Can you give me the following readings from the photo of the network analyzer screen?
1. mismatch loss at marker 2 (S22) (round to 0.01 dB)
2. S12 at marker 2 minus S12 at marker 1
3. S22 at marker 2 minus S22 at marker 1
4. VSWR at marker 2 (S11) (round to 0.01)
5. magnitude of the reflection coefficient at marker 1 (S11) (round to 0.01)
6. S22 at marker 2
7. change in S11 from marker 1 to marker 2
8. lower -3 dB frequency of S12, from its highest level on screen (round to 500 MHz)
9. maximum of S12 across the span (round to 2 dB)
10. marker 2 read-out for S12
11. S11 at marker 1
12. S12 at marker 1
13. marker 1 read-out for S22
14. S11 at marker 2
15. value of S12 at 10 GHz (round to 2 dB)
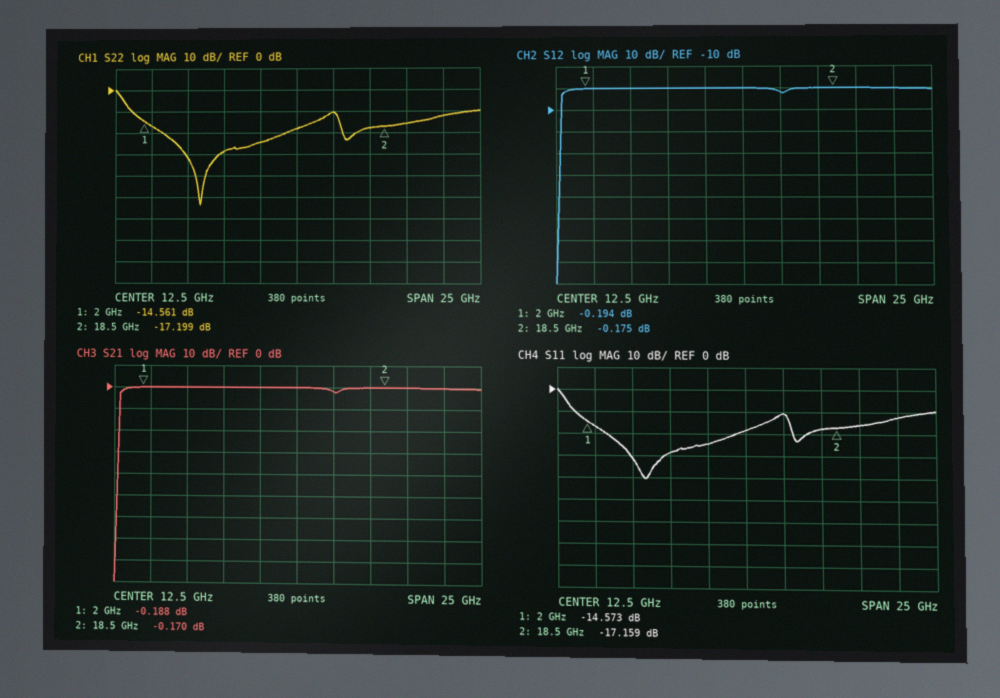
0.08 dB
0.019 dB
-2.638 dB
1.32
0.19
-17.199 dB
-2.586 dB
500 MHz
0 dB
-0.175 dB
-14.573 dB
-0.194 dB
-14.561 dB
-17.159 dB
0 dB
